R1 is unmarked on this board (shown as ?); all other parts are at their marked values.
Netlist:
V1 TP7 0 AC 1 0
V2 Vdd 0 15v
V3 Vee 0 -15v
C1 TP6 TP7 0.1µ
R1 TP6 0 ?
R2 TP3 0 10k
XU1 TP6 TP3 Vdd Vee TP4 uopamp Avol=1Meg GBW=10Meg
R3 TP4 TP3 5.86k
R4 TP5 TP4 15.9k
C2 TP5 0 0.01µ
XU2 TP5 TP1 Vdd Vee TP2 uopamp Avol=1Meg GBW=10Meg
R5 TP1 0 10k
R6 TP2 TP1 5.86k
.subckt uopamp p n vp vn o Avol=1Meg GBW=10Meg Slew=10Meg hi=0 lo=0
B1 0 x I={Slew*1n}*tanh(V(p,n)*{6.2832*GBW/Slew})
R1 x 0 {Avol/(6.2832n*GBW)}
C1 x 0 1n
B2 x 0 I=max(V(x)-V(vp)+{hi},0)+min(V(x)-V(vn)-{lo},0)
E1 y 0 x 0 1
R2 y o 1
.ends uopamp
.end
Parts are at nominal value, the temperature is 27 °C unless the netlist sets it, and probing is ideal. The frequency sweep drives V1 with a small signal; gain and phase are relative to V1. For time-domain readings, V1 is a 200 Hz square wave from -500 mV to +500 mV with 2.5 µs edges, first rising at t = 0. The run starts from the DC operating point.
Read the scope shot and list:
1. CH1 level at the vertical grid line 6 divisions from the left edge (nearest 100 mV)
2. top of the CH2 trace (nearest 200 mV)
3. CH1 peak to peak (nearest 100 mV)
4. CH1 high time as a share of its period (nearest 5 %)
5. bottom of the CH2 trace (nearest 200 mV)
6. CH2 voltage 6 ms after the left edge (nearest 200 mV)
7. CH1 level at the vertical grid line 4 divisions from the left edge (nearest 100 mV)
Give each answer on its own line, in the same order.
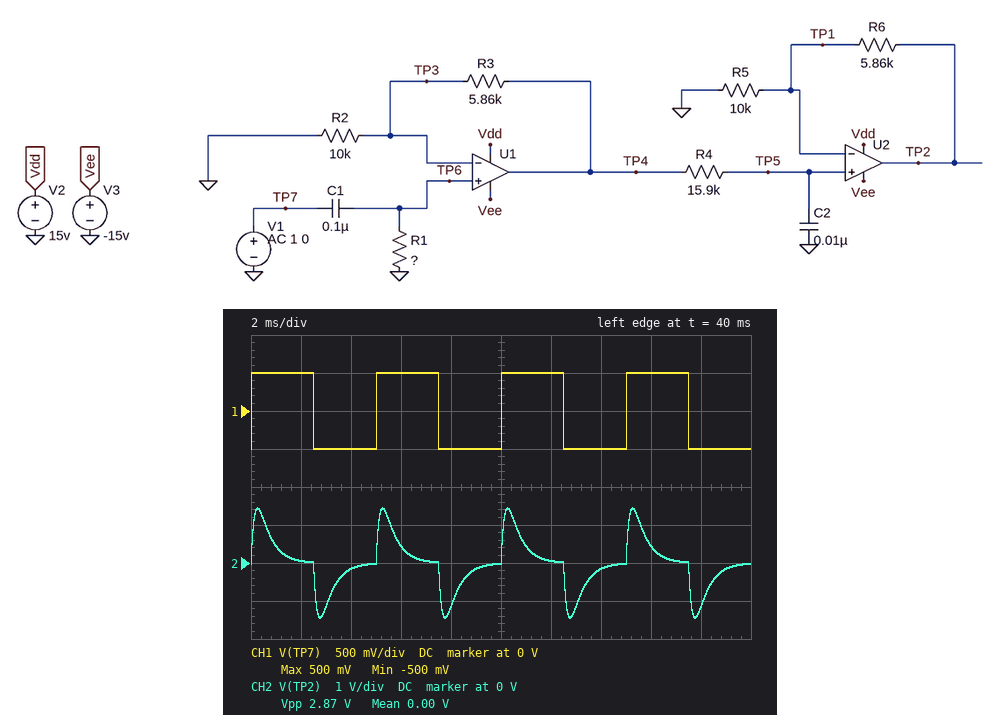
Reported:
500 mV
1.4 V
1.0 V
50 %
-1.4 V
400 mV
-500 mV
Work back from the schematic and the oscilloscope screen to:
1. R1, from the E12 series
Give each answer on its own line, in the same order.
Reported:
4.7 kΩ
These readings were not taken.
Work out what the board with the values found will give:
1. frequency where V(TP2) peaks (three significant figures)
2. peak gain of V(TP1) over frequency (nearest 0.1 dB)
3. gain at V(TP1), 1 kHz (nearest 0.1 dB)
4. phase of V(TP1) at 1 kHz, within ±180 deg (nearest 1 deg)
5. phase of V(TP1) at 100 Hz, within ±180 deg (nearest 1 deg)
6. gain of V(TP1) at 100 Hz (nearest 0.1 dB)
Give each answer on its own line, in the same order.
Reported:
582 Hz
1.5 dB
0.5 dB
-26 deg
68 deg
-7.0 dB
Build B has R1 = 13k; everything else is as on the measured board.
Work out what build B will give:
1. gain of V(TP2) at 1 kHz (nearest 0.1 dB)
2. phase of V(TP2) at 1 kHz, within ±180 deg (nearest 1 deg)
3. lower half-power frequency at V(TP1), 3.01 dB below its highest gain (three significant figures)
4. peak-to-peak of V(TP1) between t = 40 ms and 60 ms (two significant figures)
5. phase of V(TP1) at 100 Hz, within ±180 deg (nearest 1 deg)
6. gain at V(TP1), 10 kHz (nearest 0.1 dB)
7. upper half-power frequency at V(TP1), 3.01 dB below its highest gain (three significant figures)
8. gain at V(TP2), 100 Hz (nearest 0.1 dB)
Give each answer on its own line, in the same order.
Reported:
4.9 dB
-38 deg
100 Hz
2.0 V
45 deg
-16.0 dB
1.22 kHz
4.0 dB
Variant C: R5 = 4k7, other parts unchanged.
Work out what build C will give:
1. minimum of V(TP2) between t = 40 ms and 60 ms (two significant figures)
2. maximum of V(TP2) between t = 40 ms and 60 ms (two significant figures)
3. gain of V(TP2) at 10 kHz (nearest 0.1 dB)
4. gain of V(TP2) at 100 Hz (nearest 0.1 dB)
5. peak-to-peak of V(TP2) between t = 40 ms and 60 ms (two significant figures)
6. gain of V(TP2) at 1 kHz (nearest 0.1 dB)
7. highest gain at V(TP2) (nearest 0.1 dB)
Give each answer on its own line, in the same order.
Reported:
-2.0 V
2.0 V
-9.0 dB
0 dB
4.1 V
7.6 dB
8.5 dB
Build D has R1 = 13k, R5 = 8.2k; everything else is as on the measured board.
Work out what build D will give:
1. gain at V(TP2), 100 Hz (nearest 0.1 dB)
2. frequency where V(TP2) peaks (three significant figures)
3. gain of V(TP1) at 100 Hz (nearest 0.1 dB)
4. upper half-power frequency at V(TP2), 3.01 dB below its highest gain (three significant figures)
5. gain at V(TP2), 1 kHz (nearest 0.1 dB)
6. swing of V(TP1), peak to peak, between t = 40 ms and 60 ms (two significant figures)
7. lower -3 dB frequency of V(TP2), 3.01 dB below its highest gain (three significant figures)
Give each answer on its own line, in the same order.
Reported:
4.7 dB
350 Hz
0 dB
1.22 kHz
5.6 dB
2.0 V
100 Hz
